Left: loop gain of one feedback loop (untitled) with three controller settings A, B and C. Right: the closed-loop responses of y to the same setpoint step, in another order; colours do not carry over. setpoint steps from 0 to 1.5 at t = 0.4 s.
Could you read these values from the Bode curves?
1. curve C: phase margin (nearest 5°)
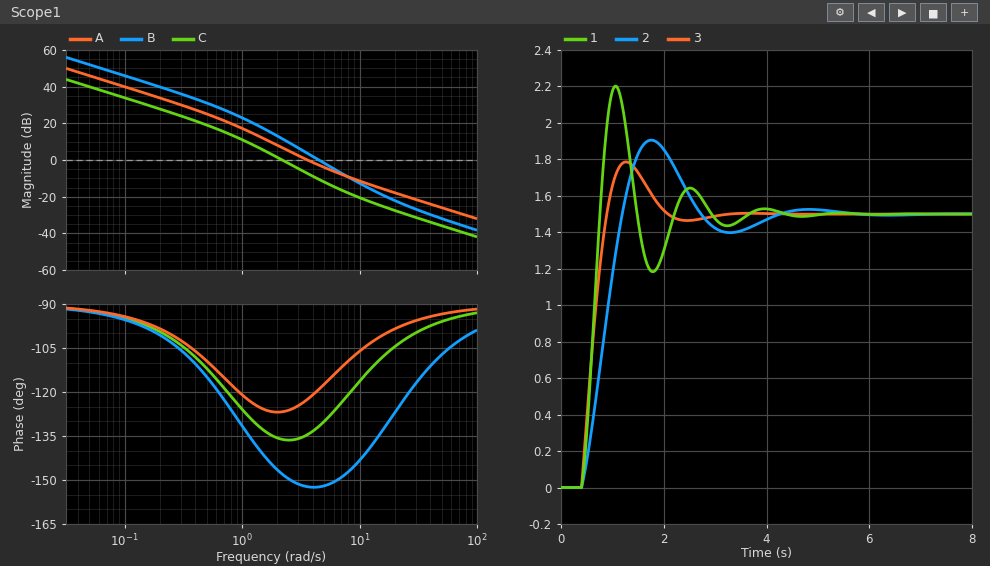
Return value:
45°
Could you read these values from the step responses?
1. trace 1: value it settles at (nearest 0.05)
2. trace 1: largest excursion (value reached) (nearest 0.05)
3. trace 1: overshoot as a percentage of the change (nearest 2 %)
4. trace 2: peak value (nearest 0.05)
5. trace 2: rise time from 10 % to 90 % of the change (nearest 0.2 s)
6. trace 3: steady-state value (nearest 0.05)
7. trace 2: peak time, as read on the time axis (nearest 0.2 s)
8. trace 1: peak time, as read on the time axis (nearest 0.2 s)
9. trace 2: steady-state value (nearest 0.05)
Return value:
1.50
2.20
46 %
1.90
0.6 s
1.50
1.8 s
1.0 s
1.50
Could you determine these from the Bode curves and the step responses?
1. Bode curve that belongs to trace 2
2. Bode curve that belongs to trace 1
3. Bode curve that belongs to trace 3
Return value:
C
B
A
